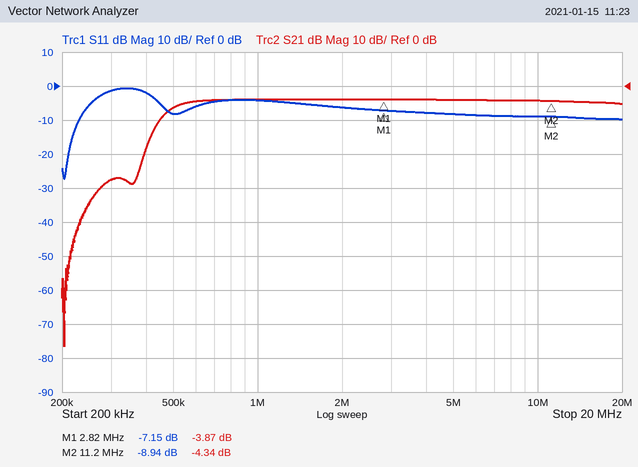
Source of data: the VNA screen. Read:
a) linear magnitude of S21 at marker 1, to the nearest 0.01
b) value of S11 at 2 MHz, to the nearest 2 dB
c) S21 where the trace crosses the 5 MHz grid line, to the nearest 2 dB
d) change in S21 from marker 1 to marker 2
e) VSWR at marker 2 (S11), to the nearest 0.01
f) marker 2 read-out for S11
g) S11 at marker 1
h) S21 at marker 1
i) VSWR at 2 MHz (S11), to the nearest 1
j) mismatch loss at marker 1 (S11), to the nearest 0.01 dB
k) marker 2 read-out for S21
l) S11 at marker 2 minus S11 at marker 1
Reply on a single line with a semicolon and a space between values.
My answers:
0.64; -6 dB; -4 dB; -0.47 dB; 2.11; -8.94 dB; -7.15 dB; -3.87 dB; 3; 0.93 dB; -4.34 dB; -1.79 dB
